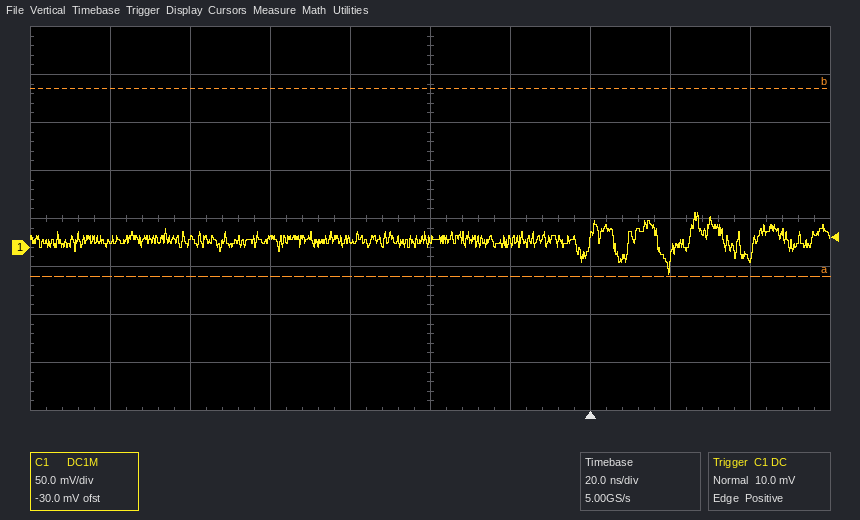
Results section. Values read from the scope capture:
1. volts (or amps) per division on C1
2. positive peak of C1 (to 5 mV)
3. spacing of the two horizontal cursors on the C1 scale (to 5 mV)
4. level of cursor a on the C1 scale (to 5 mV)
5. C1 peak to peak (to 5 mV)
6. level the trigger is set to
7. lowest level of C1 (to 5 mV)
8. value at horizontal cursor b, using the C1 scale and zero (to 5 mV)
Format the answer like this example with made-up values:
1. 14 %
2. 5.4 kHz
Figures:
1. 50 mV
2. 35 mV
3. 195 mV
4. -30 mV
5. 65 mV
6. 10.0 mV
7. -30 mV
8. 165 mV
